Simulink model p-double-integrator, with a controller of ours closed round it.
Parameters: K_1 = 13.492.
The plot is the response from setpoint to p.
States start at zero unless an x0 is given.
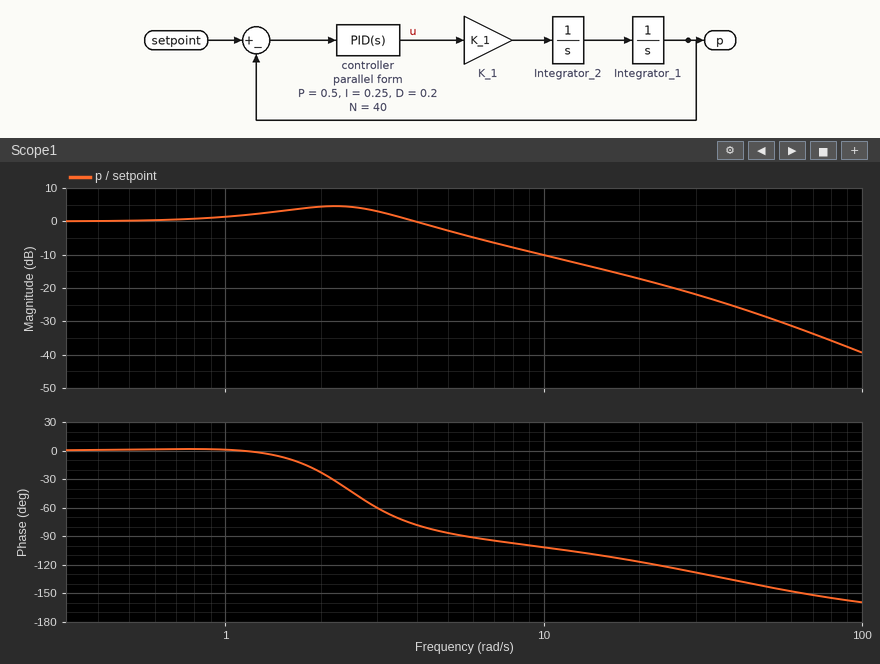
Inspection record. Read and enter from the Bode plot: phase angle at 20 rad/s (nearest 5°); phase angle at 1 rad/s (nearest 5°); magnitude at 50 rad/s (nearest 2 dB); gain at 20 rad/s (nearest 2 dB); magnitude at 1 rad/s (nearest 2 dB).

-115°
0°
-28 dB
-18 dB
2 dB
